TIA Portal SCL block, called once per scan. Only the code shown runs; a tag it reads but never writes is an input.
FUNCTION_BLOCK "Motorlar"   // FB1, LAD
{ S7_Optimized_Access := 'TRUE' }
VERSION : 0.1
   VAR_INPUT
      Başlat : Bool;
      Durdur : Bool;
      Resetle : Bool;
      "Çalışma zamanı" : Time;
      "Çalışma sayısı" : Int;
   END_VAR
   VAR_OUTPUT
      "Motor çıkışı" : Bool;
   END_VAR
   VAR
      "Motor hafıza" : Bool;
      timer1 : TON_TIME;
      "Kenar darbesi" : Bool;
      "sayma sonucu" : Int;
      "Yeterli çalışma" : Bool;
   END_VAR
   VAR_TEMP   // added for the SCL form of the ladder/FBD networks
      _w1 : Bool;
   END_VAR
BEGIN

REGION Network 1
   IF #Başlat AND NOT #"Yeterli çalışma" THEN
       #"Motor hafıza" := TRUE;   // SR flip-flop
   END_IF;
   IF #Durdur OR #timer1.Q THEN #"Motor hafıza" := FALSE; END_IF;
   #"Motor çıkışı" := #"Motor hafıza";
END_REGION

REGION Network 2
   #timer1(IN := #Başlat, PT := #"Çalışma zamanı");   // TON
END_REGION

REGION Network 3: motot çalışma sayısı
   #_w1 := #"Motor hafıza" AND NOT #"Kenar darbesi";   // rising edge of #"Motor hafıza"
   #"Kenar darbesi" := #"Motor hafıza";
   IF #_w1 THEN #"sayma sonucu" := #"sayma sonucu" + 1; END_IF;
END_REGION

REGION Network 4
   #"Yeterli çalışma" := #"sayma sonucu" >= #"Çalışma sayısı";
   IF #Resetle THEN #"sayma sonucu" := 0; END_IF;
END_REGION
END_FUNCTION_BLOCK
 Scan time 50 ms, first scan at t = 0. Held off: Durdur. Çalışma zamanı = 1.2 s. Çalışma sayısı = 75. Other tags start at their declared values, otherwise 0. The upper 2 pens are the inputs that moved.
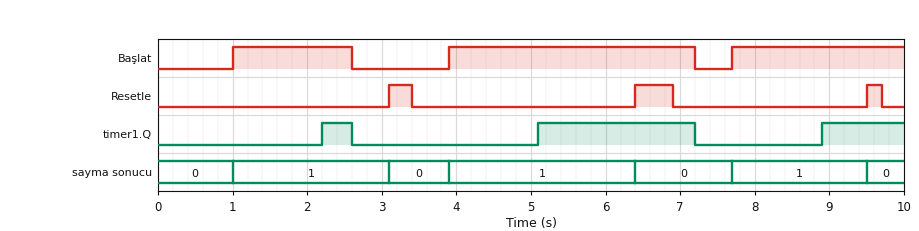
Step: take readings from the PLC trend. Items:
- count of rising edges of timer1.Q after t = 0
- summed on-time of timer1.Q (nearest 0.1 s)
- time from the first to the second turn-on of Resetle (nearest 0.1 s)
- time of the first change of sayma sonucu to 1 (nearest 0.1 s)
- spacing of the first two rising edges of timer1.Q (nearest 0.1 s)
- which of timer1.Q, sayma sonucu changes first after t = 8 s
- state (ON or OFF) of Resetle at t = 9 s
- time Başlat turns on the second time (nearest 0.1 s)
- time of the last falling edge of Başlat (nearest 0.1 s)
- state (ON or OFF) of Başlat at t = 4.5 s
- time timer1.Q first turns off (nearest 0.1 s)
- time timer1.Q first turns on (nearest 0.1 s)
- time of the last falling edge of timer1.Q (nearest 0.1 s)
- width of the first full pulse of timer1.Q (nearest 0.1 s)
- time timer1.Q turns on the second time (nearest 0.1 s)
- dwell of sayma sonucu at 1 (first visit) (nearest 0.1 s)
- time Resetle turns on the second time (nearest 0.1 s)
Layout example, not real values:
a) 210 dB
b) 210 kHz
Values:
a) 3
b) 3.6 s
c) 3.3 s
d) 1.0 s
e) 2.9 s
f) timer1.Q
g) OFF
h) 3.9 s
i) 7.2 s
j) ON
k) 2.6 s
l) 2.2 s
m) 7.2 s
n) 0.4 s
o) 5.1 s
p) 2.1 s
q) 6.4 s
